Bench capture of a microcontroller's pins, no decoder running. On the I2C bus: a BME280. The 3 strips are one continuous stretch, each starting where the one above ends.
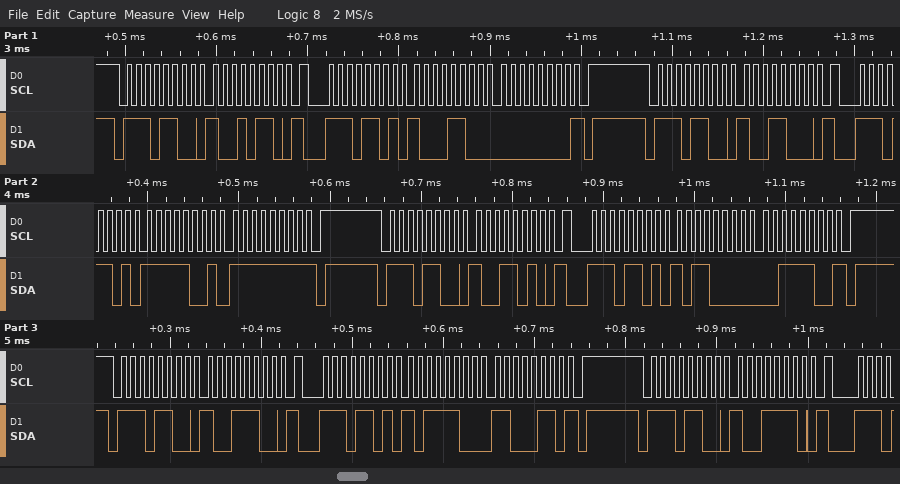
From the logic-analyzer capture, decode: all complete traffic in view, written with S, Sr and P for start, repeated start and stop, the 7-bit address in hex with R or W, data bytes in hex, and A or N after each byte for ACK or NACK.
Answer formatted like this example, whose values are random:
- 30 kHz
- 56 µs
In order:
- S 76W A 96 A Sr 76R A 8C A 00 N P S 76W A 98 A Sr 76R A F9 A FF N P S 76W A 9A A Sr 76R A B0 A 3C N P S 76W A 9C A Sr 76R A BC A C6 N P S 76W A 9E A
